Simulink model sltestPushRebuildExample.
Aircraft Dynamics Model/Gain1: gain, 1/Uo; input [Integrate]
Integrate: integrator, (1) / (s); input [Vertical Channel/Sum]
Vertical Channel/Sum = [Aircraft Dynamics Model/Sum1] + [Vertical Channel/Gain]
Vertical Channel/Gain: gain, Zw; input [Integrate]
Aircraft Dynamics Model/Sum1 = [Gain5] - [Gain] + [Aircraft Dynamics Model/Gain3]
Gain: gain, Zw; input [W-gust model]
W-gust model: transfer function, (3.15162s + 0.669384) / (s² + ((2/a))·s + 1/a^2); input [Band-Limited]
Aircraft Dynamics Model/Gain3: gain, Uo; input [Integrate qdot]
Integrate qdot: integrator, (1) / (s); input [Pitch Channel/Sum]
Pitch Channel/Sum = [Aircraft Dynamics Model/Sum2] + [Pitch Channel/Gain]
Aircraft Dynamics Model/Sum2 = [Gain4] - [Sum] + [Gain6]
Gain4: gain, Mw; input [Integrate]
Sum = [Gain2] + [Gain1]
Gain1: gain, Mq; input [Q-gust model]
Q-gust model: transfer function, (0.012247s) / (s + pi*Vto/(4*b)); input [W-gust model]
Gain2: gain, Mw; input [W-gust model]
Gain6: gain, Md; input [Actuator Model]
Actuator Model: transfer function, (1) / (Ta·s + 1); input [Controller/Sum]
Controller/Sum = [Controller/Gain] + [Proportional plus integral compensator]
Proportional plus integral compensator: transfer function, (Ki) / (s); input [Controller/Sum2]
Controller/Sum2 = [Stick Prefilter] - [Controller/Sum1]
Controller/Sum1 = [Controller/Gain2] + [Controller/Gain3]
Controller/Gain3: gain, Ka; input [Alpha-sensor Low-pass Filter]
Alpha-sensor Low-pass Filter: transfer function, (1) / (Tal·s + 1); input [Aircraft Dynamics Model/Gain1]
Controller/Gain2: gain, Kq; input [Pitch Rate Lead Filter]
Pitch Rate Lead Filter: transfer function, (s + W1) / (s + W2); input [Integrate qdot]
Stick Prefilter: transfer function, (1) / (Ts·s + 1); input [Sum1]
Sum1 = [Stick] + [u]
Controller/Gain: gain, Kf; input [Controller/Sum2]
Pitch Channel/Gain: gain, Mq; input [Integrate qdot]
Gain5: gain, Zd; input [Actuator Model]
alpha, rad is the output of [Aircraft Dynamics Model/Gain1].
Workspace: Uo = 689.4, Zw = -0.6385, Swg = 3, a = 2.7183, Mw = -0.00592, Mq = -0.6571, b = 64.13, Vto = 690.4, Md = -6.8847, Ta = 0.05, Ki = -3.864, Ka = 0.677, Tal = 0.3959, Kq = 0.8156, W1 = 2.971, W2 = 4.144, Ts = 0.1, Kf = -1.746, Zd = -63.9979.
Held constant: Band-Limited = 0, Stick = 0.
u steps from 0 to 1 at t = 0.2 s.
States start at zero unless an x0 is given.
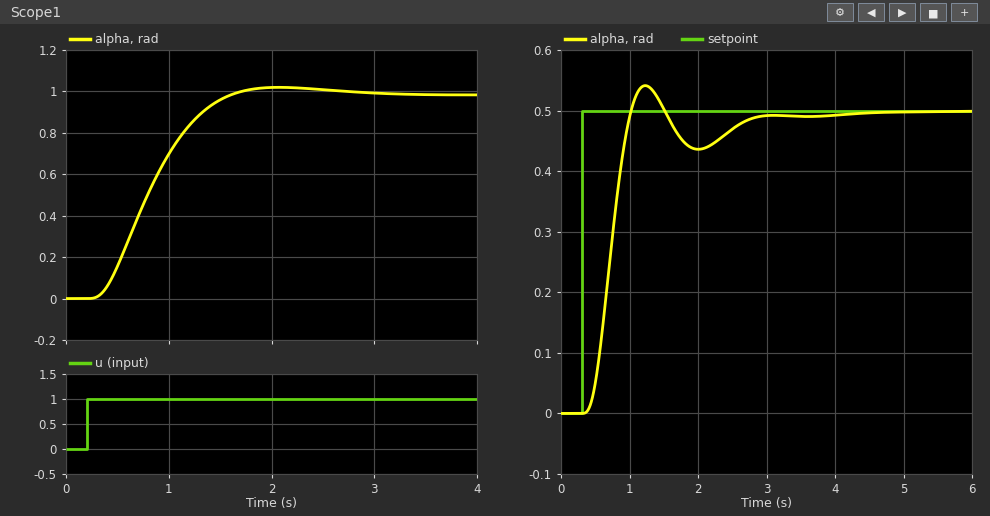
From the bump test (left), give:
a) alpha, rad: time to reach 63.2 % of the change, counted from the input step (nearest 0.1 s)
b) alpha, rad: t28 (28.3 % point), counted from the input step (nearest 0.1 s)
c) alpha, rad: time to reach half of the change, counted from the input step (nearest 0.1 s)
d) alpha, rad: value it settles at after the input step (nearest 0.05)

0.7 s
0.4 s
0.6 s
1.00
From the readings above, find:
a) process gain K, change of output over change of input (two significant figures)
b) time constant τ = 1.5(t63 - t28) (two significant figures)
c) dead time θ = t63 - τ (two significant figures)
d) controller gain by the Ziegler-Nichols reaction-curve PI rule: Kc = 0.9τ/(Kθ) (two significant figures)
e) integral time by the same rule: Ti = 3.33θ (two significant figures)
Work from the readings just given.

1.0
0.45 s
0.25 s
1.6
0.83 s
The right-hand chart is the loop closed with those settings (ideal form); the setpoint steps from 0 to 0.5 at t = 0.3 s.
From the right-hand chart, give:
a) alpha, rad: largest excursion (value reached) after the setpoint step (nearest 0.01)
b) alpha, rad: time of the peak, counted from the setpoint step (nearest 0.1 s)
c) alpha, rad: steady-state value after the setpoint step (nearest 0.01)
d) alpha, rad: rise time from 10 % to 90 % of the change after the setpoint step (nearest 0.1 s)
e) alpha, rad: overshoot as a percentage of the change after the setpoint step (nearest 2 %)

0.54
0.9 s
0.50
0.4 s
8 %
